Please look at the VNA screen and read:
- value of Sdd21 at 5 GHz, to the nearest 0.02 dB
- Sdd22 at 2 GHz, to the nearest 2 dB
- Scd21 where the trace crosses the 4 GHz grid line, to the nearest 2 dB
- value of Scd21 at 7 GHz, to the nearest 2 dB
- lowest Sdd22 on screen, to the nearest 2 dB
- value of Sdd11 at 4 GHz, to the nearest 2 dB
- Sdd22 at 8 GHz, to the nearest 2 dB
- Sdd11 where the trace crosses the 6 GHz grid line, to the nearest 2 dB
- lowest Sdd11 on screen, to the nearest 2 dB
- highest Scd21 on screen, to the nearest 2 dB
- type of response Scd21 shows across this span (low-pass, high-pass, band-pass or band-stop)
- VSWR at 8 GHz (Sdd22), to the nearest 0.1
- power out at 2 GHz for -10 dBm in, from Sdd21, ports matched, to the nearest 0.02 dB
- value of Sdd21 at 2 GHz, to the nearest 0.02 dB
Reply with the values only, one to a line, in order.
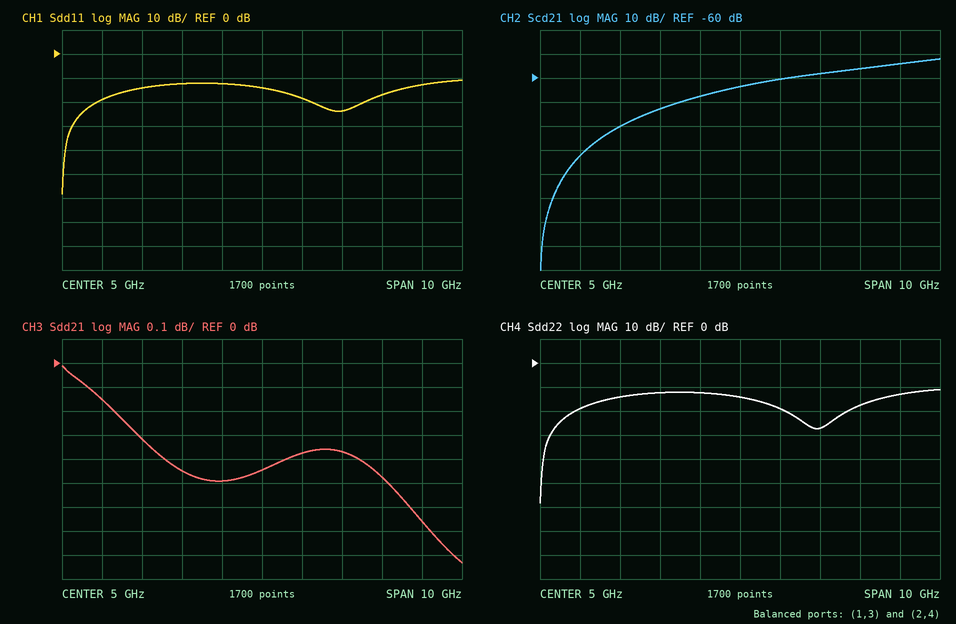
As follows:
-0.44 dB
-14 dB
-68 dB
-58 dB
-58 dB
-12 dB
-18 dB
-18 dB
-58 dB
-52 dB
high-pass
1.3
-10.32 dBm
-0.32 dB
